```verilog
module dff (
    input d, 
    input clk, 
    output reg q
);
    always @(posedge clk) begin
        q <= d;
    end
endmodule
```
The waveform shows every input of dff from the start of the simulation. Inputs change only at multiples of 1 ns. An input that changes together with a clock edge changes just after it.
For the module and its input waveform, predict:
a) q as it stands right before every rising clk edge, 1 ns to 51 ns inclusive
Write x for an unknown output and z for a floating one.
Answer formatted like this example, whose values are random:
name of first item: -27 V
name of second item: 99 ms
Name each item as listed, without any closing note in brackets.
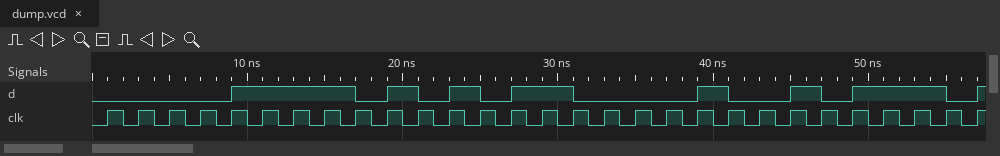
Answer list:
q as it stands right before every rising clk edge, 1 ns to 51 ns inclusive: x 0 0 0 0 0 1 1 1 1 0 1 0 1 0 1 1 0 0 0 0 1 0 0 1 0
